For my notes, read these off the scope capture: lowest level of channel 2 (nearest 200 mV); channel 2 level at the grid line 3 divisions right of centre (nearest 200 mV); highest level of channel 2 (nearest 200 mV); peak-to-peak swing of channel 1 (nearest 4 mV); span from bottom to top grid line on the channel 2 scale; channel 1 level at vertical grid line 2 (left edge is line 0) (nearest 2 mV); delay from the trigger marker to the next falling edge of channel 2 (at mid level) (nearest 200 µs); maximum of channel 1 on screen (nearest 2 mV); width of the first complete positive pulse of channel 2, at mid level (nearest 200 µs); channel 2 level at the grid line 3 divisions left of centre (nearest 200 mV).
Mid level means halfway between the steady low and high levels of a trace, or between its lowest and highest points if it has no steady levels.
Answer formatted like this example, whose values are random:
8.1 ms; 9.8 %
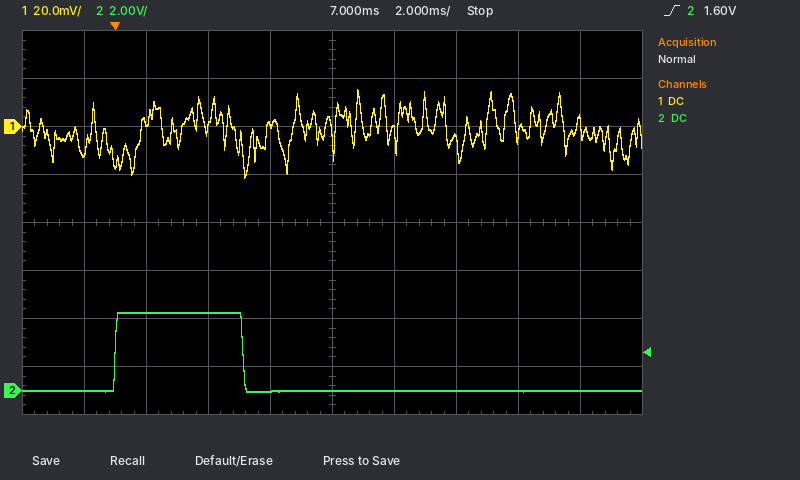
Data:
0.0 V; 0.0 V; 3.2 V; 36 mV; 16 V; 2 mV; 4.2 ms; 16 mV; 4.2 ms; 3.2 V
